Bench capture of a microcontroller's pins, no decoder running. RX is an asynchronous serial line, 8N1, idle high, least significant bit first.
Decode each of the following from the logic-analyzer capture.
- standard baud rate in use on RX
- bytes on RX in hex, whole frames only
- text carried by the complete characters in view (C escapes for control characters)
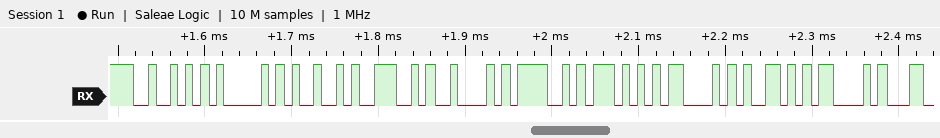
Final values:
115200 baud
0x52 0x41 0x49 0x4E 0x42 0x4F 0x57 0x43 0x59 0x43
"RAINBOWCYC"
